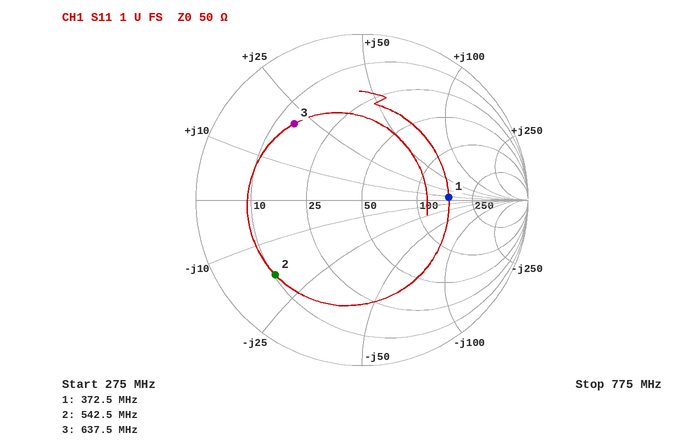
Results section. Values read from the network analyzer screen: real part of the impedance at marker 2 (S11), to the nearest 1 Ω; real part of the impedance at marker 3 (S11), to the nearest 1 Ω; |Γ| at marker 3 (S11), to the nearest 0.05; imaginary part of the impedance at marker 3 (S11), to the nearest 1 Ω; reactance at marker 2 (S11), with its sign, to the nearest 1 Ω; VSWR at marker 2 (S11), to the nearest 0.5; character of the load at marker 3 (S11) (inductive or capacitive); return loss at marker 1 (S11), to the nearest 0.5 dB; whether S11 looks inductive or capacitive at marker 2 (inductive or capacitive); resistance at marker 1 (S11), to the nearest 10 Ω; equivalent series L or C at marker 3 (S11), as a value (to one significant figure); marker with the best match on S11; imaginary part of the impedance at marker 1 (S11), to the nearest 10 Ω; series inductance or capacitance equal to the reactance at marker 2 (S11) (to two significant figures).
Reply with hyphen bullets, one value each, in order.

- 10 Ω
- 14 Ω
- 0.60
- +21 Ω
- -18 Ω
- 5.5
- inductive
- 5.5 dB
- capacitive
- 160 Ω
- 5 nH
- marker 1
- +10 Ω
- 16 pF
